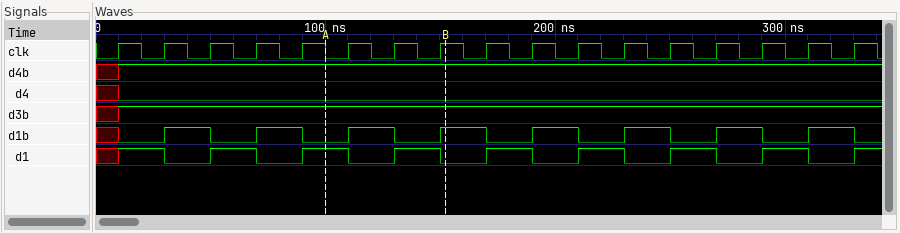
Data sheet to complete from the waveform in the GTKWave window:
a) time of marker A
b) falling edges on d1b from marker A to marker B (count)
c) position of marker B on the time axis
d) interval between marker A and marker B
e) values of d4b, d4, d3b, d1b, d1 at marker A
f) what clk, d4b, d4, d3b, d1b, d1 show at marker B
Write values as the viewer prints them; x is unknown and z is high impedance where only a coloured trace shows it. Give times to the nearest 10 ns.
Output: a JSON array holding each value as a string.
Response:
["100 ns", "1", "150 ns", "50 ns", "d4b=1, d4=0, d3b=1, d1b=0, d1=1", "clk=1, d4b=1, d4=0, d3b=1, d1b=1, d1=0"]
